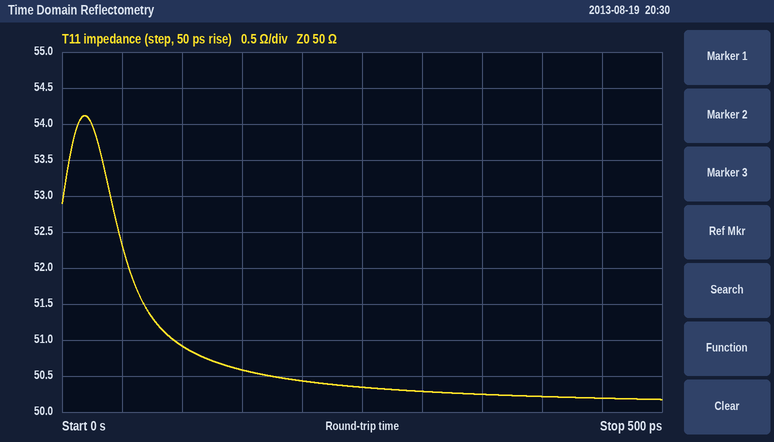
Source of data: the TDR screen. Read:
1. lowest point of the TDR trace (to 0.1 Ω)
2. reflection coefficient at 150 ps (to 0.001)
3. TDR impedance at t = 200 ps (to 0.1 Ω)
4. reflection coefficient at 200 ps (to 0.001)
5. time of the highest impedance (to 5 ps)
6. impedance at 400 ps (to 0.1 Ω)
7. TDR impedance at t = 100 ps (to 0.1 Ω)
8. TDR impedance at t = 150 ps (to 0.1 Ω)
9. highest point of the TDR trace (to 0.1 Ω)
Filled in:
50.2 Ω
+0.006
50.4 Ω
+0.004
20 ps
50.2 Ω
50.9 Ω
50.6 Ω
54.1 Ω
